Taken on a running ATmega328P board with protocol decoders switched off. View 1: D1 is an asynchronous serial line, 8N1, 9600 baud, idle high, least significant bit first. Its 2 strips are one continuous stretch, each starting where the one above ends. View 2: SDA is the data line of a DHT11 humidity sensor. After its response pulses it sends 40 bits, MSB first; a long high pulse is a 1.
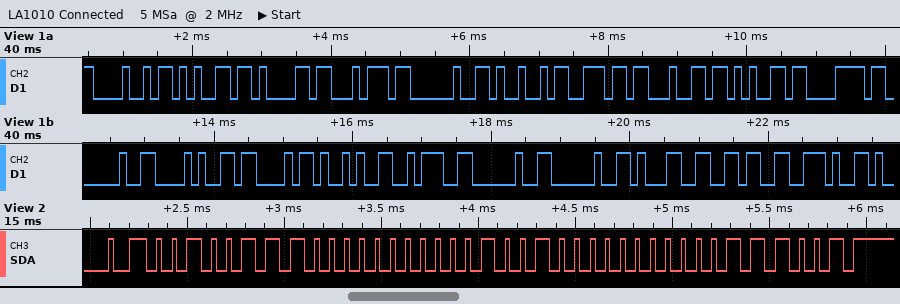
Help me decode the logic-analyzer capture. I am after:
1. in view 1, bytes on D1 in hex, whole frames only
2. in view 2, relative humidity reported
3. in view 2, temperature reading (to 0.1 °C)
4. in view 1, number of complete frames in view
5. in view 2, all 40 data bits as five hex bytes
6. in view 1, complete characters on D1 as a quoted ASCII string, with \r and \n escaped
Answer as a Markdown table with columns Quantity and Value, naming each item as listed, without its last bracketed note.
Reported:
| Quantity | Value |
|---|---|
| in view 1, bytes on D1 in hex, whole frames only | 48 65 61 74 20 49 6E 64 65 78 20 28 43 29 3A 20 20 31 36 2E |
| in view 2, relative humidity reported | 39 % |
| in view 2, temperature reading | 18.0 °C |
| in view 1, number of complete frames in view | 20 |
| in view 2, all 40 data bits as five hex bytes | 27 00 12 00 39 |
| in view 1, complete characters on D1 as a quoted ASCII string, with \r and \n escaped | "Heat Index (C):  16." |
